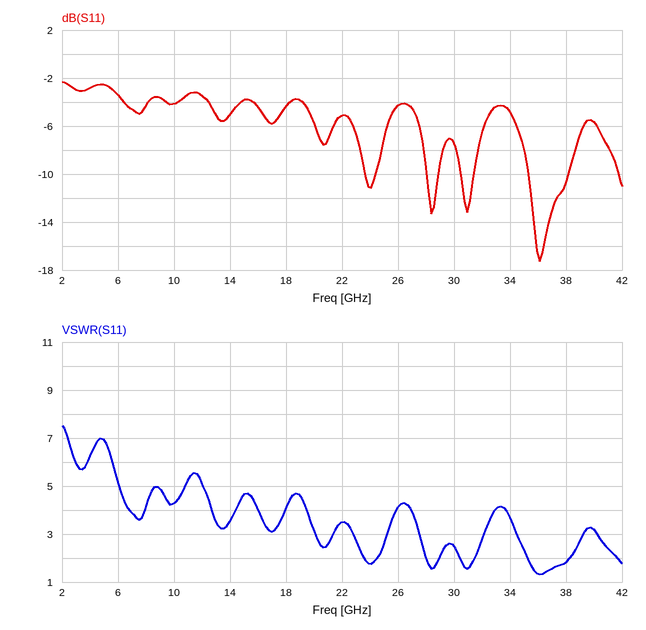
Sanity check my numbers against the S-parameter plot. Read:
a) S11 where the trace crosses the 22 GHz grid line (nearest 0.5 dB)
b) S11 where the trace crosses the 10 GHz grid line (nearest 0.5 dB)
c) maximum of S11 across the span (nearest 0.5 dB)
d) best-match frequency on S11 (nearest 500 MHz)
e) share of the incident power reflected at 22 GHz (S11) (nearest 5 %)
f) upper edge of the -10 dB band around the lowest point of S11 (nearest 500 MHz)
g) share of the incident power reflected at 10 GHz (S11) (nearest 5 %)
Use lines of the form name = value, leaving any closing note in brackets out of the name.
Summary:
S11 where the trace crosses the 22 GHz grid line = -5.0 dB
S11 where the trace crosses the 10 GHz grid line = -4.0 dB
maximum of S11 across the span = -2.5 dB
best-match frequency on S11 = 36.0 GHz
share of the incident power reflected at 22 GHz (S11) = 30 %
upper edge of the -10 dB band around the lowest point of S11 = 38.0 GHz
share of the incident power reflected at 10 GHz (S11) = 40 %
